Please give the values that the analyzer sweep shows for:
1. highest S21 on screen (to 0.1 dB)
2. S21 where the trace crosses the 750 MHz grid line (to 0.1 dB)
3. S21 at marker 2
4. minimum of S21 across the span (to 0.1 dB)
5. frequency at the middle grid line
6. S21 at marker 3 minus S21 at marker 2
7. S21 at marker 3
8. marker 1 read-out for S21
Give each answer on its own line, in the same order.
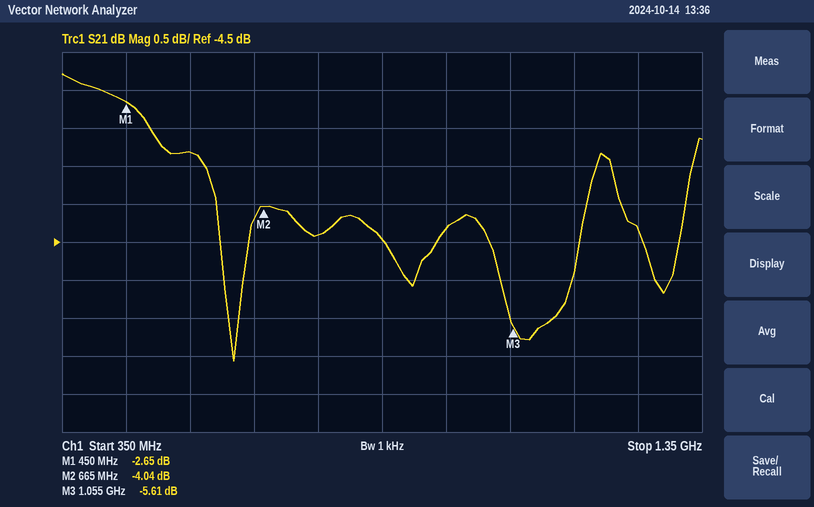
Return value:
-2.3 dB
-4.4 dB
-4.04 dB
-6.1 dB
850 MHz
-1.57 dB
-5.61 dB
-2.65 dB
